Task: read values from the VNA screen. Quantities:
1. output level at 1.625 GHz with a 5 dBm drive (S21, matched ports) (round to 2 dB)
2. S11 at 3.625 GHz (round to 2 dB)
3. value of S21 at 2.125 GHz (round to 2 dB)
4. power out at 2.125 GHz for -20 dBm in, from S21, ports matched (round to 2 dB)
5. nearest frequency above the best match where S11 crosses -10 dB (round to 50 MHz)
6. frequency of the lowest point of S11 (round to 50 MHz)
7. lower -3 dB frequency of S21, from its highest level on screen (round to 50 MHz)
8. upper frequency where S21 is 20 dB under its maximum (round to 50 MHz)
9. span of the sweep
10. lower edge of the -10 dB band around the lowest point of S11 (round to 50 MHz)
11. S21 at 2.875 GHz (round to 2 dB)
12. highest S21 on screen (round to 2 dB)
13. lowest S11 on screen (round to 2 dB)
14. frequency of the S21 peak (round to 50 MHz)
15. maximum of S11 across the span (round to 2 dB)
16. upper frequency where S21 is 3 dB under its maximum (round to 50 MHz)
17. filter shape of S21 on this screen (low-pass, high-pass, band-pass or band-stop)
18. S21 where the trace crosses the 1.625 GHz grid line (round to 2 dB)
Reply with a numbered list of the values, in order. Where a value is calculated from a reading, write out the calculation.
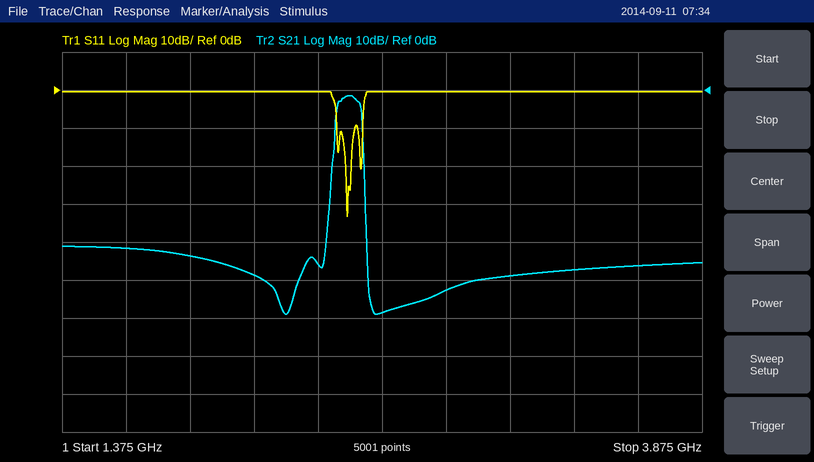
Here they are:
1. 5 dBm + (-42 dB) = -36 dBm
2. 0 dB
3. -48 dB
4. -20 dBm + (-48 dB) = -68 dBm
5. 2.50 GHz
6. 2.50 GHz
7. 2.45 GHz
8. 2.55 GHz
9. 2.5 GHz
10. 2.45 GHz
11. -52 dB
12. -2 dB
13. -34 dB
14. 2.50 GHz
15. 0 dB
16. 2.55 GHz
17. band-pass
18. -42 dB
